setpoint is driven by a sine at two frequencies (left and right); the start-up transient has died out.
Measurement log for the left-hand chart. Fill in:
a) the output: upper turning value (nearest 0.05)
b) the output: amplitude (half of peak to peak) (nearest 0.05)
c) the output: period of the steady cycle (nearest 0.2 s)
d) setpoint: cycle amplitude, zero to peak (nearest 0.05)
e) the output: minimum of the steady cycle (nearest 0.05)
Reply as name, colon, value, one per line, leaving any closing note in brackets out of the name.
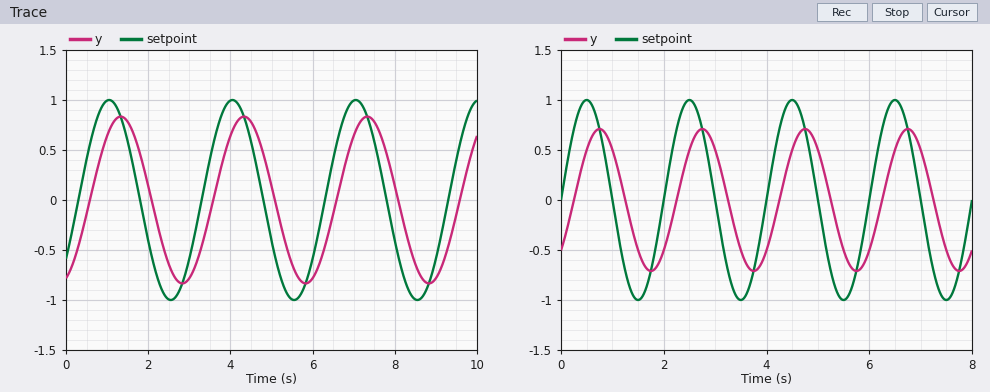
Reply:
the output: upper turning value: 0.85
the output: amplitude (half of peak to peak): 0.85
the output: period of the steady cycle: 3.0 s
setpoint: cycle amplitude, zero to peak: 1.00
the output: minimum of the steady cycle: -0.85
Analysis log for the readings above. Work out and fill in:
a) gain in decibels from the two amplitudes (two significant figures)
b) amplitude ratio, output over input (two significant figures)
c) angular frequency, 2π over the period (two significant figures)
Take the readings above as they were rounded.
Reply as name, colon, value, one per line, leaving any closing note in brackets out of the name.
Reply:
gain in decibels from the two amplitudes: -1.4 dB
amplitude ratio, output over input: 0.85
angular frequency, 2π over the period: 2.1 rad/s
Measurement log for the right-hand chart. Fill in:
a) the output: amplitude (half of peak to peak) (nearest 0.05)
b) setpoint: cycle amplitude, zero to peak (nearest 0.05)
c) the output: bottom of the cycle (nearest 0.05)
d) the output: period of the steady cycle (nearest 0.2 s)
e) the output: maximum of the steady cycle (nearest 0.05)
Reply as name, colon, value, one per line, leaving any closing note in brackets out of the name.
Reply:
the output: amplitude (half of peak to peak): 0.70
setpoint: cycle amplitude, zero to peak: 1.00
the output: bottom of the cycle: -0.70
the output: period of the steady cycle: 2.0 s
the output: maximum of the steady cycle: 0.70
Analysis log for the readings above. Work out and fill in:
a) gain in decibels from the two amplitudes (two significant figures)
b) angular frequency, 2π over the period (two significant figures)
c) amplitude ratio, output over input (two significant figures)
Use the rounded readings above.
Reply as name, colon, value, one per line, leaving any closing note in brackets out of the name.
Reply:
gain in decibels from the two amplitudes: -3.1 dB
angular frequency, 2π over the period: 3.1 rad/s
amplitude ratio, output over input: 0.70
